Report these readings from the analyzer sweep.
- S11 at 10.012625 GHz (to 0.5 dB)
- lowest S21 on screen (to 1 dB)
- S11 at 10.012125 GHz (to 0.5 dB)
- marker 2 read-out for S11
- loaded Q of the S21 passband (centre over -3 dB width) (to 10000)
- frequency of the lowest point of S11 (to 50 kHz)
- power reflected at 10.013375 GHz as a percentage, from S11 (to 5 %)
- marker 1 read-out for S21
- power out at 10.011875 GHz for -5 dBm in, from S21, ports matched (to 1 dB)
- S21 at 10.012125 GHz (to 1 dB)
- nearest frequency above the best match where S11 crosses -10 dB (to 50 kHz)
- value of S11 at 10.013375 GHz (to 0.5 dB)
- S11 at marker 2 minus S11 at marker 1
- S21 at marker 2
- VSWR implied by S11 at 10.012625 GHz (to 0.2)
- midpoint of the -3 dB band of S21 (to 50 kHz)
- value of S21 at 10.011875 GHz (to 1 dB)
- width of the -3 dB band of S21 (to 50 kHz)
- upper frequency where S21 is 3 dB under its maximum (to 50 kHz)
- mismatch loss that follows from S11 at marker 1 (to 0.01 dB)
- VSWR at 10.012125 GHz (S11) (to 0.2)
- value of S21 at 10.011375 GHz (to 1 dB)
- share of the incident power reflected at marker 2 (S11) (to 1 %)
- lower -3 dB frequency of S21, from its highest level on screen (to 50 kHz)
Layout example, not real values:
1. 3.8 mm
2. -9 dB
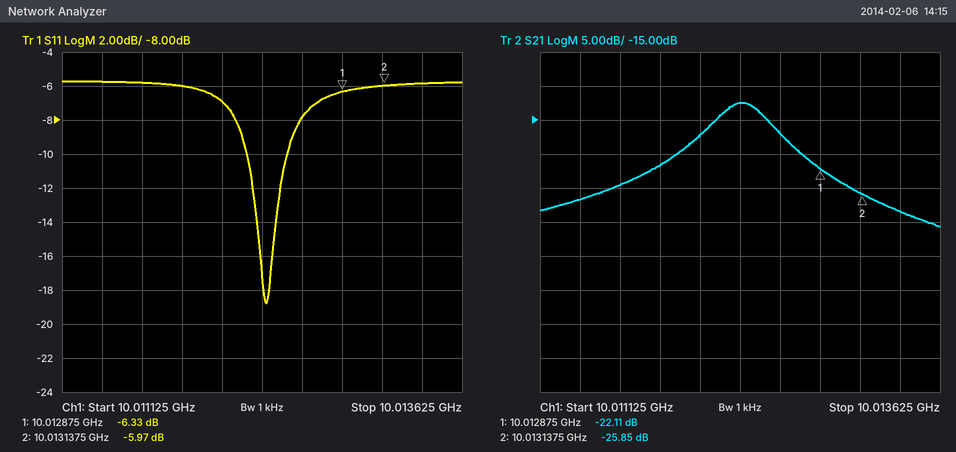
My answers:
1. -8.0 dB
2. -31 dB
3. -7.0 dB
4. -5.97 dB
5. 30000
6. 10.01240 GHz
7. 25 %
8. -22.11 dB
9. -27 dBm
10. -17 dB
11. 10.01255 GHz
12. -6.0 dB
13. 0.36 dB
14. -25.85 dB
15. 2.4
16. 10.01240 GHz
17. -22 dB
18. 350 kHz
19. 10.01255 GHz
20. 1.15 dB
21. 2.6
22. -27 dB
23. 25 %
24. 10.01220 GHz
